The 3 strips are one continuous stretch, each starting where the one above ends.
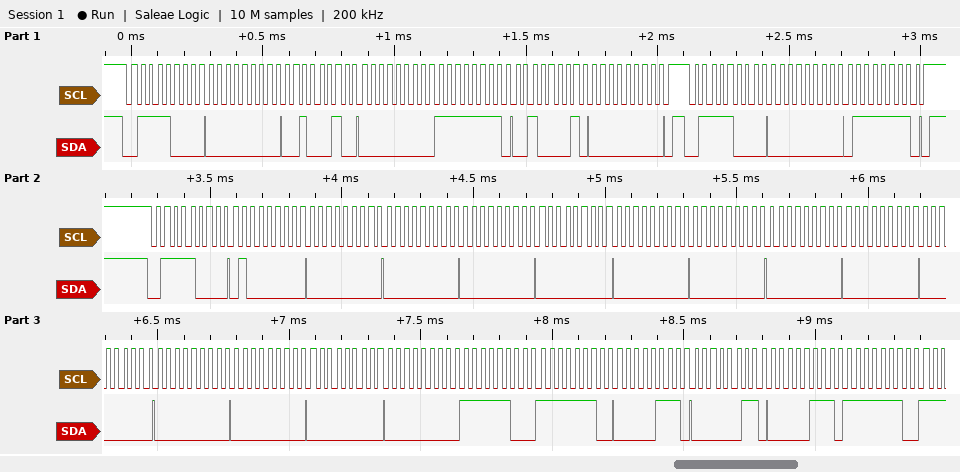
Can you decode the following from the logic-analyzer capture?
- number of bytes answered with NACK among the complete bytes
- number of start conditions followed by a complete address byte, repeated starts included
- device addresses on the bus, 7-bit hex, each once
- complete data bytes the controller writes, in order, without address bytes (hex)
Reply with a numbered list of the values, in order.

1. 0
2. 3
3. 0x3C
4. 00 22 00 FF 21 00 00 7F 40 00 00 00 00 00 00 00 00 00 00 00 00 00 FC FE 07 03 07 FE
